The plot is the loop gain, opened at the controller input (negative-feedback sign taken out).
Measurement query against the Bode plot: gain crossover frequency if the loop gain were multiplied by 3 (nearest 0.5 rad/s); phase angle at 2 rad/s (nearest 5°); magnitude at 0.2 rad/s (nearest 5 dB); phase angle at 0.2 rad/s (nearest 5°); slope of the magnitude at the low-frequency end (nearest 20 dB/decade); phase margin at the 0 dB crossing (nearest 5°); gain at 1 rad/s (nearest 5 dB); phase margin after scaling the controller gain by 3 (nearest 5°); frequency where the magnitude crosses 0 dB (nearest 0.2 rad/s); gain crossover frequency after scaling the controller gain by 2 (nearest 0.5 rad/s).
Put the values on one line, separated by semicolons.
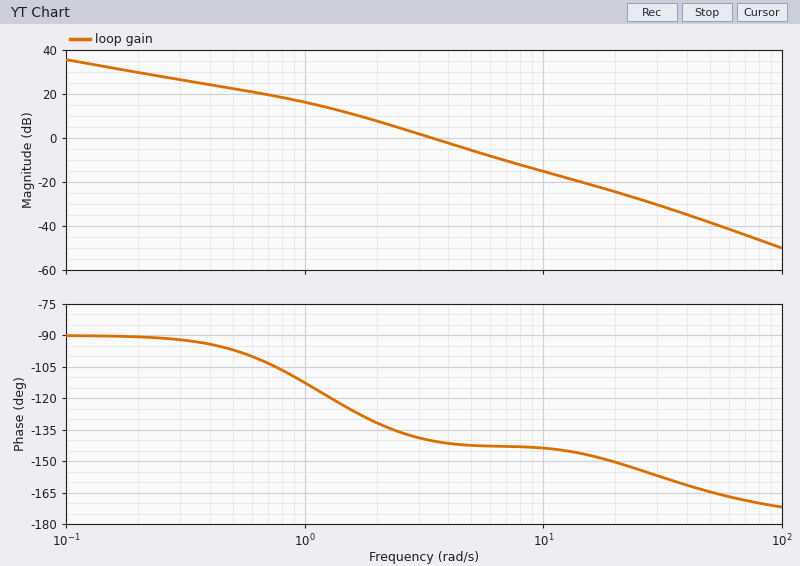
6.5 rad/s; -130°; 30 dB; -90°; -20 dB/decade; 40°; 15 dB; 35°; 3.4 rad/s; 5.0 rad/s
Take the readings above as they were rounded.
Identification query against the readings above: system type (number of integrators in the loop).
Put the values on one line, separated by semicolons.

1
